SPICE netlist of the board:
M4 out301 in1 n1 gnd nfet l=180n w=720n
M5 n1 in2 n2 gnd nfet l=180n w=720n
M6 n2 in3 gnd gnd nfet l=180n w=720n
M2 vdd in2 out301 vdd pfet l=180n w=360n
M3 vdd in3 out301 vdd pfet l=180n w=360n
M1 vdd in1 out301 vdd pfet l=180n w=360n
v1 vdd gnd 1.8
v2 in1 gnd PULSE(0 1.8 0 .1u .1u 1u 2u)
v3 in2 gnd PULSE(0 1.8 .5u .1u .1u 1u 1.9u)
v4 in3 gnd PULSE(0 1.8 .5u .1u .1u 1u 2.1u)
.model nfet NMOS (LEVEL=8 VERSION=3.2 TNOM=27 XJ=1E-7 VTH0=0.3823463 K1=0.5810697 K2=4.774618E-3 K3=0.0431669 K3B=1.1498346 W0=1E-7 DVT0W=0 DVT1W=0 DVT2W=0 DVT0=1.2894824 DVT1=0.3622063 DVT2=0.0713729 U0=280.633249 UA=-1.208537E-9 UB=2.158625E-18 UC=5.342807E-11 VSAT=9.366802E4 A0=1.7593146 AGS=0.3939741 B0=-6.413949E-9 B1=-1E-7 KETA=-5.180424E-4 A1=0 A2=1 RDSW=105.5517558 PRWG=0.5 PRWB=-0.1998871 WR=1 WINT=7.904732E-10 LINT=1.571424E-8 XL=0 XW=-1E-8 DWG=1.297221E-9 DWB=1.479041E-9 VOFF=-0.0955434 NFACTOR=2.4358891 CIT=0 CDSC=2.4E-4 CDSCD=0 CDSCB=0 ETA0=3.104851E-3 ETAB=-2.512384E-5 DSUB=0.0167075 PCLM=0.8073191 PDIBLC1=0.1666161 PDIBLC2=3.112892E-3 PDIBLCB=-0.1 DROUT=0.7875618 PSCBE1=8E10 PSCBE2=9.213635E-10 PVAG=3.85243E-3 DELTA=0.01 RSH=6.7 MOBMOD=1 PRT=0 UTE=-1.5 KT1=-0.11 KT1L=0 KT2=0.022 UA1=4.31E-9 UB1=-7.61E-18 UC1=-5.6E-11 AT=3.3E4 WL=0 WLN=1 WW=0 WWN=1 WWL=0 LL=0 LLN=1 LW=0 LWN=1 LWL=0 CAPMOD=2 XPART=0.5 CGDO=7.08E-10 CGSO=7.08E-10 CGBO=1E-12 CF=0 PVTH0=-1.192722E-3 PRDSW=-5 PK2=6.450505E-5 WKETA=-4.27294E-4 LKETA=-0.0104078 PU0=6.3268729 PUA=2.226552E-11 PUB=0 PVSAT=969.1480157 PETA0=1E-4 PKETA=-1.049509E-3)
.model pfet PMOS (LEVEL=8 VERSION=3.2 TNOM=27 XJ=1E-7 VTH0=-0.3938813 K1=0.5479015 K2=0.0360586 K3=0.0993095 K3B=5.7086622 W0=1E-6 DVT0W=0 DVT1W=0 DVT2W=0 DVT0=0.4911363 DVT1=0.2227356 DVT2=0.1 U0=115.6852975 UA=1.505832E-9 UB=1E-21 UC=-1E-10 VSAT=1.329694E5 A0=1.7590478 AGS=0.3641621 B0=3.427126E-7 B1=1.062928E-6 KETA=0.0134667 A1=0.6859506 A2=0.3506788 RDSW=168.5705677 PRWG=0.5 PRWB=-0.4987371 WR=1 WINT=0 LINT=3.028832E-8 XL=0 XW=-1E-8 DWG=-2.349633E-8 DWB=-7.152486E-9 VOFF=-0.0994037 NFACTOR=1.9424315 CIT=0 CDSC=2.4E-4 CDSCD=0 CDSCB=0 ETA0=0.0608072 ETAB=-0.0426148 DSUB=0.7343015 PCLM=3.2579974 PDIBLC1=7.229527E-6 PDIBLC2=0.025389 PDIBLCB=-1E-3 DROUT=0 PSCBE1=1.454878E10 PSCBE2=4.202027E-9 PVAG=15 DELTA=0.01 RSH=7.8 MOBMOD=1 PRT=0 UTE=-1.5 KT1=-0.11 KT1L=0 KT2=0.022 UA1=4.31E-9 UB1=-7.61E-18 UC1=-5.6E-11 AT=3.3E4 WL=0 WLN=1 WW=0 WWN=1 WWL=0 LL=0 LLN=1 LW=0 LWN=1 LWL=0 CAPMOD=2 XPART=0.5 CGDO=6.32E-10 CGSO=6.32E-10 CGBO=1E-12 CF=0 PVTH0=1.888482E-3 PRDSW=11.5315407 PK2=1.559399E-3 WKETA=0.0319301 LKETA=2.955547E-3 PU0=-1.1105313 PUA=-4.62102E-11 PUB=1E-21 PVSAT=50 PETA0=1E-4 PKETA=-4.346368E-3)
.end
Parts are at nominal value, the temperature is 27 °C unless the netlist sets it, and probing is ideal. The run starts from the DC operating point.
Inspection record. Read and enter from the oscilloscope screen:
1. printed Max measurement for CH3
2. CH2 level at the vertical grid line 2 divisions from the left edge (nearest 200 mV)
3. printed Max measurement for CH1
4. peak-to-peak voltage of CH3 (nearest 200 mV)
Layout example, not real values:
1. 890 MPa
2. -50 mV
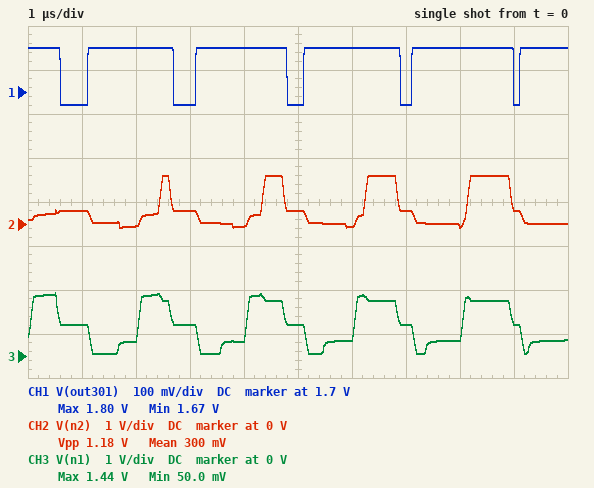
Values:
1. 1.44 V
2. 0 V
3. 1.80 V
4. 1.4 V
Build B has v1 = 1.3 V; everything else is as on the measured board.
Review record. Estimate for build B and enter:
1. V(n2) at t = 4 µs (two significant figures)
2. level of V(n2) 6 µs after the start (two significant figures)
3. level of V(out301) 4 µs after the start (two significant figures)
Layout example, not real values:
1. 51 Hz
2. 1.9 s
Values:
1. -76 mV
2. -79 mV
3. 1.3 V
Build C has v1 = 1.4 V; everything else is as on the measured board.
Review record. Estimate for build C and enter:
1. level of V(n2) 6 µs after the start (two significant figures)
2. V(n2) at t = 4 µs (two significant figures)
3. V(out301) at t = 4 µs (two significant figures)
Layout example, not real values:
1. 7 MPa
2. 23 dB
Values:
1. -77 mV
2. -73 mV
3. 1.4 V
